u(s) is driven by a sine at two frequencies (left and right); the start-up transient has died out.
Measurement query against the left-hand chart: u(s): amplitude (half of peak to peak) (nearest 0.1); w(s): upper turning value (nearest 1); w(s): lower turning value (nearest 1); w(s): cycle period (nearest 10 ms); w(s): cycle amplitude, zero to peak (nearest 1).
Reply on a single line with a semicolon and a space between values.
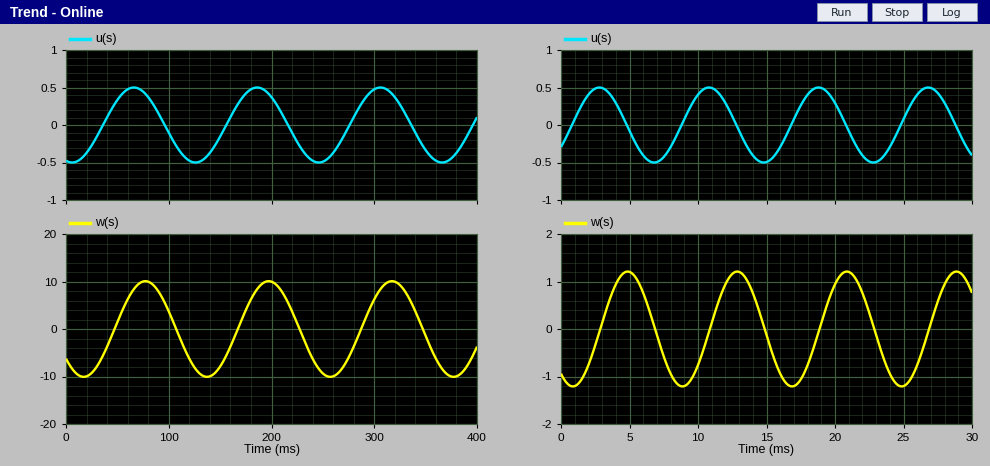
0.5; 10; -10; 120 ms; 10
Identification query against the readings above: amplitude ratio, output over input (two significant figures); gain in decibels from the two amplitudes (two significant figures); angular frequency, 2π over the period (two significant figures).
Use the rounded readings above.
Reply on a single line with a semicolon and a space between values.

20; 26 dB; 0.052 rad/ms
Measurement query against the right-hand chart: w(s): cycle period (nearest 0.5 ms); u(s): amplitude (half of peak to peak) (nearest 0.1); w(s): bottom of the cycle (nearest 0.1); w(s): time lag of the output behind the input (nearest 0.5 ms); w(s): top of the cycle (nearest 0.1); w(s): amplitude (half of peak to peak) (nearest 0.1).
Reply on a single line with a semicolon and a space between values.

8.0 ms; 0.5; -1.2; 2.0 ms; 1.2; 1.2
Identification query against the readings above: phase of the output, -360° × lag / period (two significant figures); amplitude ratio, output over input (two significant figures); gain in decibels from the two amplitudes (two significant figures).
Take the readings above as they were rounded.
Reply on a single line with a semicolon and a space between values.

-90°; 2.4; 7.6 dB
